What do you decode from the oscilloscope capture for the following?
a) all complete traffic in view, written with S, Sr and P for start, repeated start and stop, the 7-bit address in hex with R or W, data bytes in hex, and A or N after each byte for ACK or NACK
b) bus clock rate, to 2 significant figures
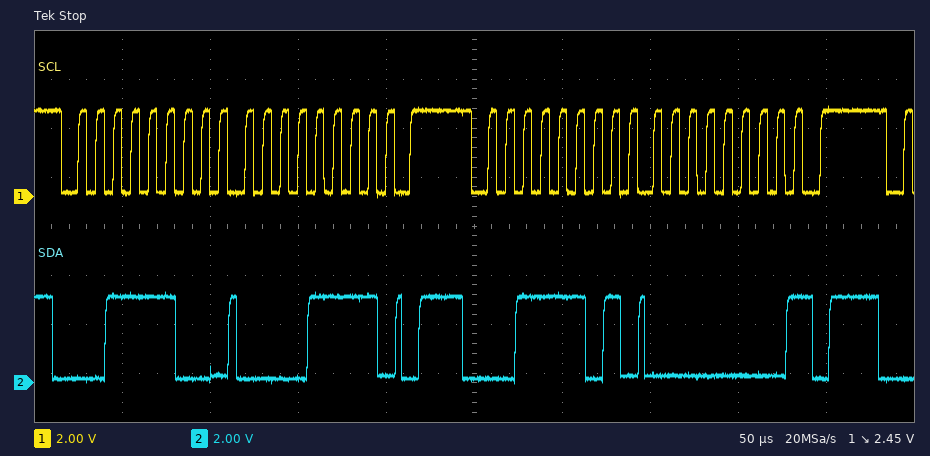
S 1EW A 0F A P S 1ER A 00 N P
100 kHz
